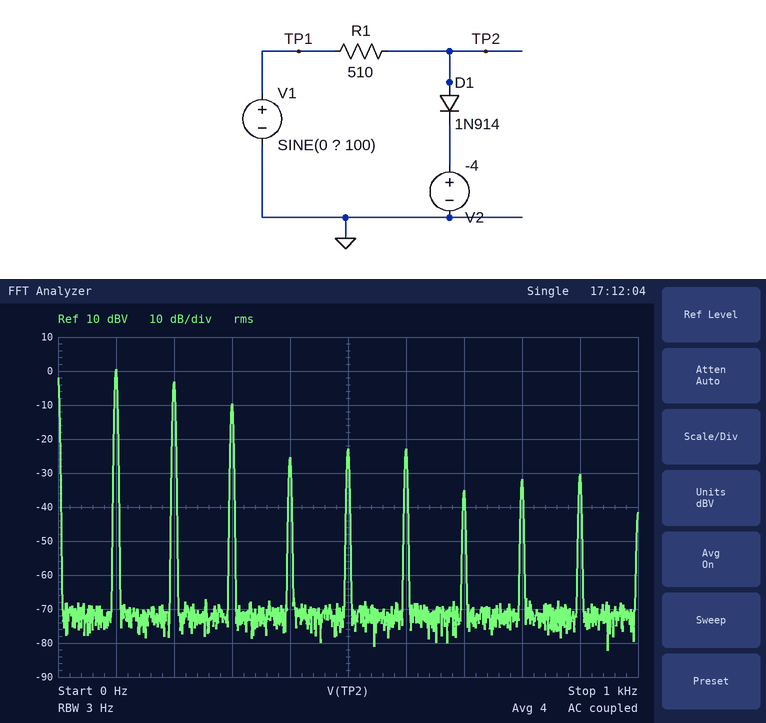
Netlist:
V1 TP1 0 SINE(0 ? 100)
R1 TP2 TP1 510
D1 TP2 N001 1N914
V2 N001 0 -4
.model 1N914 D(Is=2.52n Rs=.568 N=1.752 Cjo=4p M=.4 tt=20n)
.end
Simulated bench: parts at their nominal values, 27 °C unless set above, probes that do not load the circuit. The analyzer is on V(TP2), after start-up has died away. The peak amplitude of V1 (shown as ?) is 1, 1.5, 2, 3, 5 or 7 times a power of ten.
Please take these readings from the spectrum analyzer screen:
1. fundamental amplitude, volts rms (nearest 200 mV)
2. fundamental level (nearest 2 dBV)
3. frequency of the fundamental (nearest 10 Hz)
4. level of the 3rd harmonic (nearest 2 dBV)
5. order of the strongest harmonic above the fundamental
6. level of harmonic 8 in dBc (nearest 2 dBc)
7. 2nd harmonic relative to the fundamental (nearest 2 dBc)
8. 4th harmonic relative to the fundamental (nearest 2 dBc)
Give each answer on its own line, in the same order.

1.0 V
0 dBV
100 Hz
-10 dBV
2
-32 dBc
-4 dBc
-26 dBc
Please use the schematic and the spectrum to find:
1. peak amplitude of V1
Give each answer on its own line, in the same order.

7 V
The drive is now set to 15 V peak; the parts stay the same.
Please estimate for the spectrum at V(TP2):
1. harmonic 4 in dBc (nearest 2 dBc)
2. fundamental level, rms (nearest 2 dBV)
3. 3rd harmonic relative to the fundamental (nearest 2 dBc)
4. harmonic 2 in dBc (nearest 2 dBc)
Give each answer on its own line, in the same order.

-22 dBc
12 dBV
-18 dBc
-6 dBc
